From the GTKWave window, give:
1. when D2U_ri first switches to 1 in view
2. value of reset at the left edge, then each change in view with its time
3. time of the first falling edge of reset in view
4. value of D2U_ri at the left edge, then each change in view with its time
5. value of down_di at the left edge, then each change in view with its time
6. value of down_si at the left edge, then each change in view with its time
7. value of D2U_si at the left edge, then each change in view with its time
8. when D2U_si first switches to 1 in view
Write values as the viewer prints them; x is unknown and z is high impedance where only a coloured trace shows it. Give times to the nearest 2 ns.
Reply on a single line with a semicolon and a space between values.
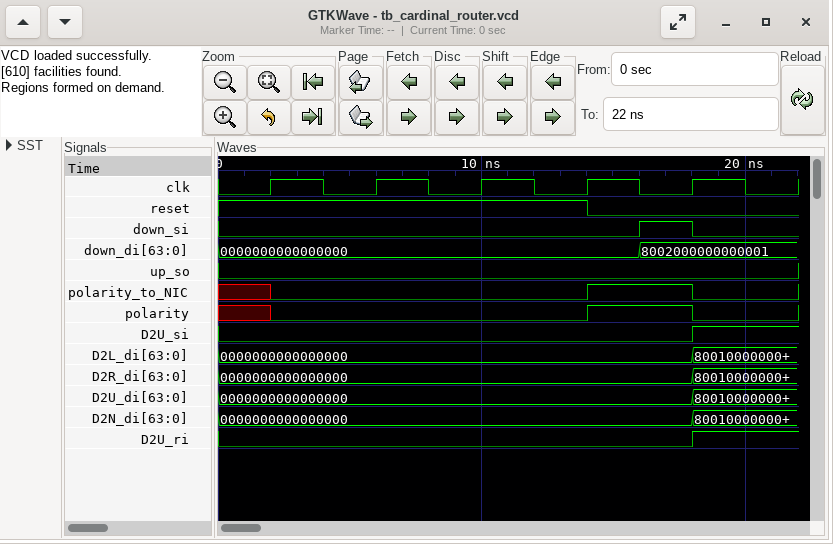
18 ns; 1, 0 at 14 ns; 14 ns; 0, 1 at 18 ns; 0000000000000000, 8002000000000001 at 16 ns; 0, 1 at 16 ns, 0 at 18 ns; 0, 1 at 18 ns; 18 ns
